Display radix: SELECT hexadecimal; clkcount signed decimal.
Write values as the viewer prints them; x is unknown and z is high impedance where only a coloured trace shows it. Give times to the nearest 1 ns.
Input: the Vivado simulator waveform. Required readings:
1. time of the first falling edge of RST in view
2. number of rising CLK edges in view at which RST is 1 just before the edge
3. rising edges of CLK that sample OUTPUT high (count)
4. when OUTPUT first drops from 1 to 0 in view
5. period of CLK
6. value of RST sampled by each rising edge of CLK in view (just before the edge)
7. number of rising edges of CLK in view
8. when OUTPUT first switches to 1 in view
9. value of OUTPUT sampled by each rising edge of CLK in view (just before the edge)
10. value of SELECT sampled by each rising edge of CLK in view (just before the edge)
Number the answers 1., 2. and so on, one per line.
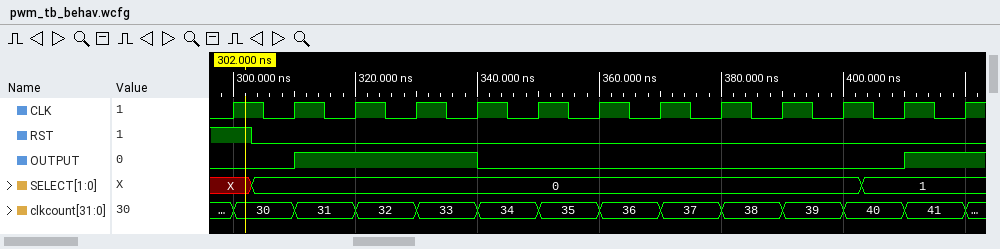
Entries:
1. 303 ns
2. 1
3. 4
4. 340 ns
5. 10 ns
6. 1 0 0 0 0 0 0 0 0 0 0 0 0
7. 13
8. 310 ns
9. 0 0 1 1 1 0 0 0 0 0 0 0 1
10. X, 0, 0, 0, 0, 0, 0, 0, 0, 0, 0, 1, 1
